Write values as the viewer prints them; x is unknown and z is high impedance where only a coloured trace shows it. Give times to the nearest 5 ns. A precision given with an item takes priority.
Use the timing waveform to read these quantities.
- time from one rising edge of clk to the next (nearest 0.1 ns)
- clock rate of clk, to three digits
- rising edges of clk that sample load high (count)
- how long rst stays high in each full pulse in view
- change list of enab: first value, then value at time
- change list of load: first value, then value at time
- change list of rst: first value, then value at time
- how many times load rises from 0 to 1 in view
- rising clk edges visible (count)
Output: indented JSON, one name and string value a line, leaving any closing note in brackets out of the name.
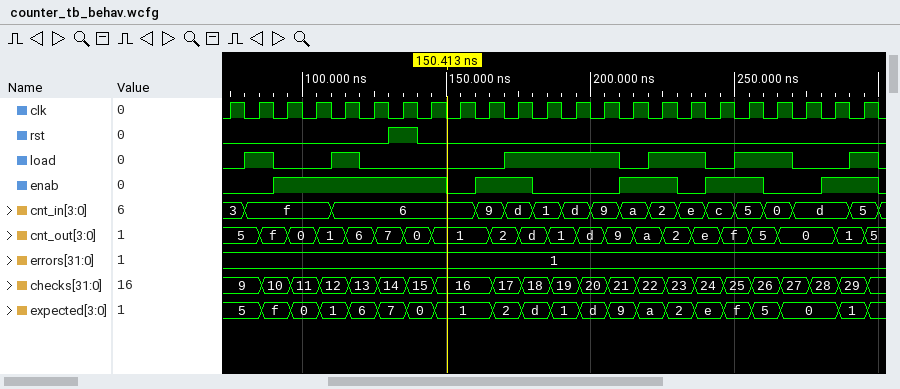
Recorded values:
{
  "time from one rising edge of clk to the next": "10 ns",
  "clock rate of clk, to three digits": "100 MHz",
  "rising edges of clk that sample load high": "11",
  "how long rst stays high in each full pulse in view": "10 ns",
  "change list of enab: first value, then value at time": "0, 1 at 90 ns, 0 at 150 ns, 1 at 160 ns, 0 at 180 ns, 1 at 210 ns, 0 at 230 ns, 1 at 240 ns, 0 at 260 ns, 1 at 280 ns, 0 at 300 ns",
  "change list of load: first value, then value at time": "0, 1 at 80 ns, 0 at 90 ns, 1 at 110 ns, 0 at 120 ns, 1 at 170 ns, 0 at 210 ns, 1 at 220 ns, 0 at 240 ns, 1 at 250 ns, 0 at 270 ns, 1 at 290 ns, 0 at 300 ns",
  "change list of rst: first value, then value at time": "0, 1 at 130 ns, 0 at 140 ns",
  "how many times load rises from 0 to 1 in view": "6",
  "rising clk edges visible": "23"
}
